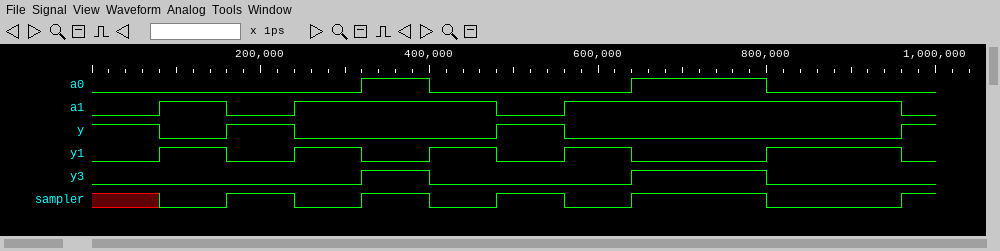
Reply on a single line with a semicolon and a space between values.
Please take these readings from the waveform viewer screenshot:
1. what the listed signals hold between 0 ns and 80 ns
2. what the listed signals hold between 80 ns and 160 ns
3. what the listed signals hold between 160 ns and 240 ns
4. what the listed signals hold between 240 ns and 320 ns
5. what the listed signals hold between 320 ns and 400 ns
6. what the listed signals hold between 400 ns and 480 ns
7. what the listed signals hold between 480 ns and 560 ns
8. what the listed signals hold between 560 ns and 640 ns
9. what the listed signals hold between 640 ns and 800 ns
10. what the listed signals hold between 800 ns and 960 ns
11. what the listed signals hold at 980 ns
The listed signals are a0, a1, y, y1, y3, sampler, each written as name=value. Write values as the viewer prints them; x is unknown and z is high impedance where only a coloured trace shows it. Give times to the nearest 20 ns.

a0=0, a1=0, y=1, y1=0, y3=0, sampler=x; a0=0, a1=1, y=0, y1=1, y3=0, sampler=0; a0=0, a1=0, y=1, y1=0, y3=0, sampler=1; a0=0, a1=1, y=0, y1=1, y3=0, sampler=0; a0=1, a1=1, y=0, y1=0, y3=1, sampler=1; a0=0, a1=1, y=0, y1=1, y3=0, sampler=0; a0=0, a1=0, y=1, y1=0, y3=0, sampler=1; a0=0, a1=1, y=0, y1=1, y3=0, sampler=0; a0=1, a1=1, y=0, y1=0, y3=1, sampler=1; a0=0, a1=1, y=0, y1=1, y3=0, sampler=0; a0=0, a1=0, y=1, y1=0, y3=0, sampler=1
